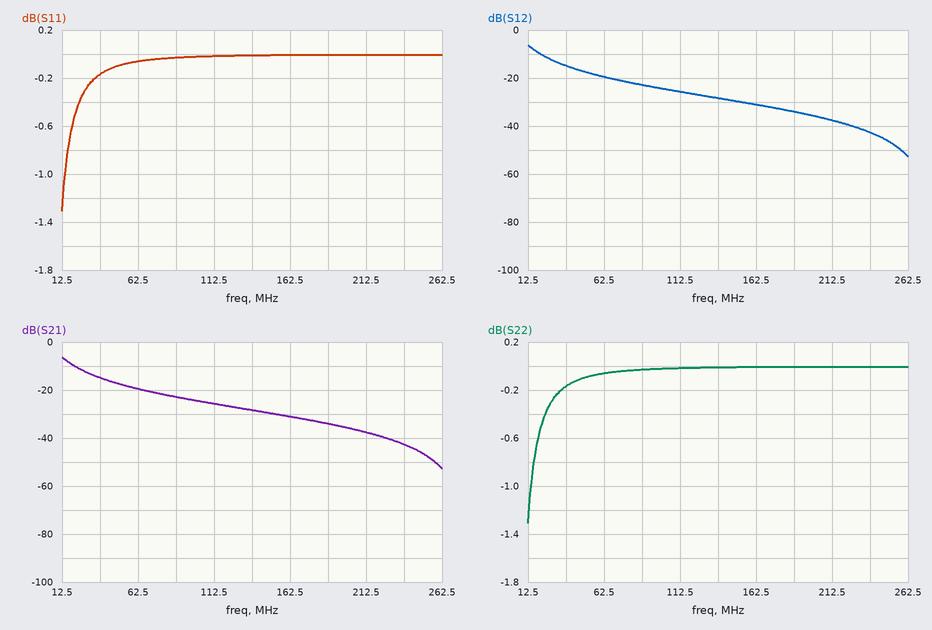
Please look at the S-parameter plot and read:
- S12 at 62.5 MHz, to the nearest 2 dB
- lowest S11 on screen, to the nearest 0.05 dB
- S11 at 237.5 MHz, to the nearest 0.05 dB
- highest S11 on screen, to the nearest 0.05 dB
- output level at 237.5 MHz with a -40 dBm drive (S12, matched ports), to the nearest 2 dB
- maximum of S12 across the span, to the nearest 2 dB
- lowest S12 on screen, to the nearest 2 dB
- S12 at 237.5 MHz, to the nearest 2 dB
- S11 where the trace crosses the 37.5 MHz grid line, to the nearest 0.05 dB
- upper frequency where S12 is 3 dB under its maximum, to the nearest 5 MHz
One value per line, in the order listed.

-20 dB
-1.30 dB
0.00 dB
0.00 dB
-82 dBm
-6 dB
-52 dB
-42 dB
-0.15 dB
20 MHz
